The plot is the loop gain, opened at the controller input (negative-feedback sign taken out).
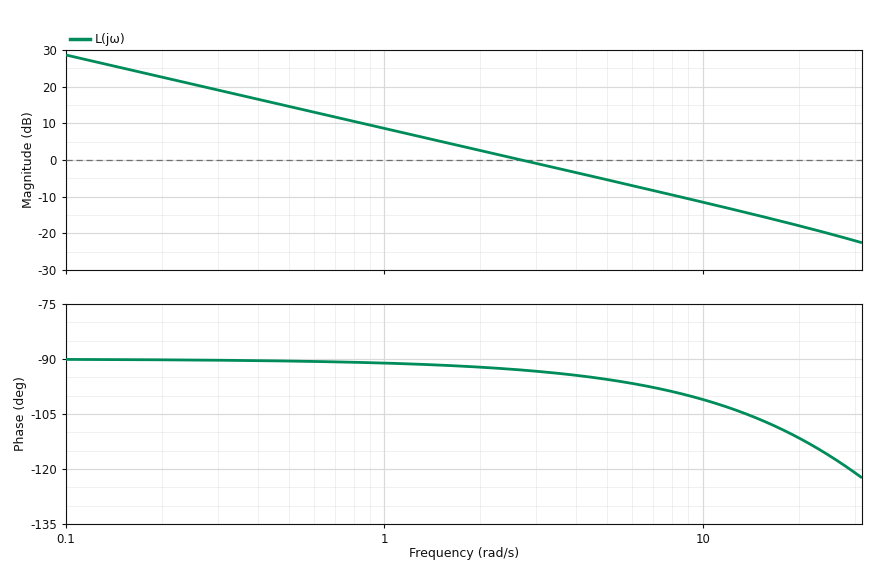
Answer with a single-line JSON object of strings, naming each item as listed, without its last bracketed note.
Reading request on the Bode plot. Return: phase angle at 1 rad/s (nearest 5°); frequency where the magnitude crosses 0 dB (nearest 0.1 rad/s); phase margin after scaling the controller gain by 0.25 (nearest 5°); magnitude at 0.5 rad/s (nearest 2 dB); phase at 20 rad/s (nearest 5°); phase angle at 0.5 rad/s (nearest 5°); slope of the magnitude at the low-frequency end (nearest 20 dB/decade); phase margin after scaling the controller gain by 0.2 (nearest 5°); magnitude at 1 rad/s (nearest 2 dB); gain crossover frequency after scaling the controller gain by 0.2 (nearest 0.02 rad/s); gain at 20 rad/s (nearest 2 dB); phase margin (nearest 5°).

{"phase angle at 1 rad/s": "-90°", "frequency where the magnitude crosses 0 dB": "2.7 rad/s", "phase margin after scaling the controller gain by 0.25": "90°", "magnitude at 0.5 rad/s": "14 dB", "phase at 20 rad/s": "-110°", "phase angle at 0.5 rad/s": "-90°", "slope of the magnitude at the low-frequency end": "-20 dB/decade", "phase margin after scaling the controller gain by 0.2": "90°", "magnitude at 1 rad/s": "8 dB", "gain crossover frequency after scaling the controller gain by 0.2": "0.54 rad/s", "gain at 20 rad/s": "-18 dB", "phase margin": "85°"}
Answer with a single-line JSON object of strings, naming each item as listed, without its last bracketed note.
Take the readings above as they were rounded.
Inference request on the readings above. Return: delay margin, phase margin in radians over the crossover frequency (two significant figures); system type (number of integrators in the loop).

{"delay margin, phase margin in radians over the crossover frequency": "0.55 s", "system type": "1"}
